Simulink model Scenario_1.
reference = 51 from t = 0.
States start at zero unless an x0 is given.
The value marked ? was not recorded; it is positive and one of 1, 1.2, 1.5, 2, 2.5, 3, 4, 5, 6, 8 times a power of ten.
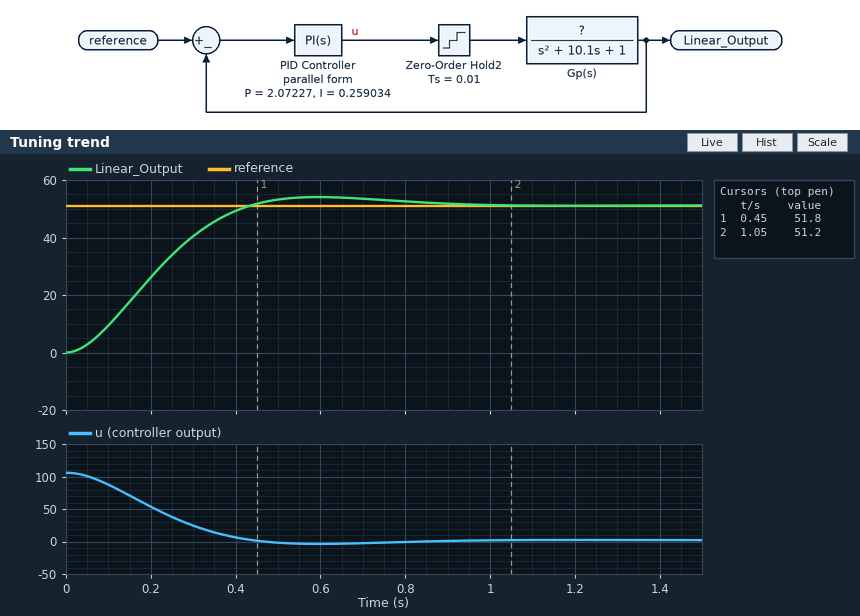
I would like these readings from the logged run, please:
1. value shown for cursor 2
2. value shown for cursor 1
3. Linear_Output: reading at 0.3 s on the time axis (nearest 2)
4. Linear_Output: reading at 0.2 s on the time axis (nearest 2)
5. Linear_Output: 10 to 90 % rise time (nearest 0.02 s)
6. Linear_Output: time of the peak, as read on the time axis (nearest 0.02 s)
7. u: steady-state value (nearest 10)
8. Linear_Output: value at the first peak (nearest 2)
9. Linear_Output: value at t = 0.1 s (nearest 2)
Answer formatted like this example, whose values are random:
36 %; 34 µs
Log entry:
51.2; 51.8; 40; 26; 0.28 s; 0.60 s; 0; 54; 10
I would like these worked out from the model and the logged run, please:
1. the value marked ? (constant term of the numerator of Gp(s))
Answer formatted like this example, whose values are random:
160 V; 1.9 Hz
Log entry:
25
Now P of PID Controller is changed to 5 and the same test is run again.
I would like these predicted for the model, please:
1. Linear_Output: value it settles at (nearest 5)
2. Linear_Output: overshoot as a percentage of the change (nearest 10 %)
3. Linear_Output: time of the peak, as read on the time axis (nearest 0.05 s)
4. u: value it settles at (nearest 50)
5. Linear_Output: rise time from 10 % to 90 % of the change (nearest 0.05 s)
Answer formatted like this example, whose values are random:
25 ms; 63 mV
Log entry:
50; 20 %; 0.30 s; 0; 0.15 s
